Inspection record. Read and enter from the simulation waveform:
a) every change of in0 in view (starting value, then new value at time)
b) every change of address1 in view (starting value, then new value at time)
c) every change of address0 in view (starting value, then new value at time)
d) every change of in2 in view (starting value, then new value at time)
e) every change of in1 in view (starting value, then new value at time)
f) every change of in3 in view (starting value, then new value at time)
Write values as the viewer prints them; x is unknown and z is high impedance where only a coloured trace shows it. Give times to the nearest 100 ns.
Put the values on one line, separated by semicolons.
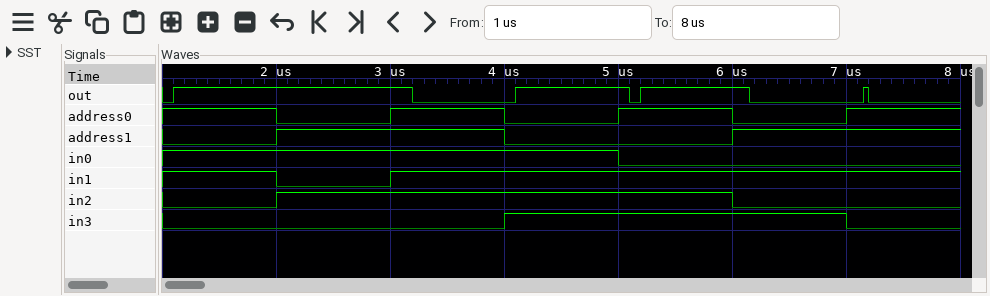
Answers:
1, 0 at 5000 ns; 0, 1 at 2000 ns, 0 at 4000 ns, 1 at 6000 ns; 1, 0 at 2000 ns, 1 at 3000 ns, 0 at 4000 ns, 1 at 5000 ns, 0 at 6000 ns, 1 at 7000 ns; 0, 1 at 2000 ns, 0 at 6000 ns; 1, 0 at 2000 ns, 1 at 3000 ns; 0, 1 at 4000 ns, 0 at 7000 ns
